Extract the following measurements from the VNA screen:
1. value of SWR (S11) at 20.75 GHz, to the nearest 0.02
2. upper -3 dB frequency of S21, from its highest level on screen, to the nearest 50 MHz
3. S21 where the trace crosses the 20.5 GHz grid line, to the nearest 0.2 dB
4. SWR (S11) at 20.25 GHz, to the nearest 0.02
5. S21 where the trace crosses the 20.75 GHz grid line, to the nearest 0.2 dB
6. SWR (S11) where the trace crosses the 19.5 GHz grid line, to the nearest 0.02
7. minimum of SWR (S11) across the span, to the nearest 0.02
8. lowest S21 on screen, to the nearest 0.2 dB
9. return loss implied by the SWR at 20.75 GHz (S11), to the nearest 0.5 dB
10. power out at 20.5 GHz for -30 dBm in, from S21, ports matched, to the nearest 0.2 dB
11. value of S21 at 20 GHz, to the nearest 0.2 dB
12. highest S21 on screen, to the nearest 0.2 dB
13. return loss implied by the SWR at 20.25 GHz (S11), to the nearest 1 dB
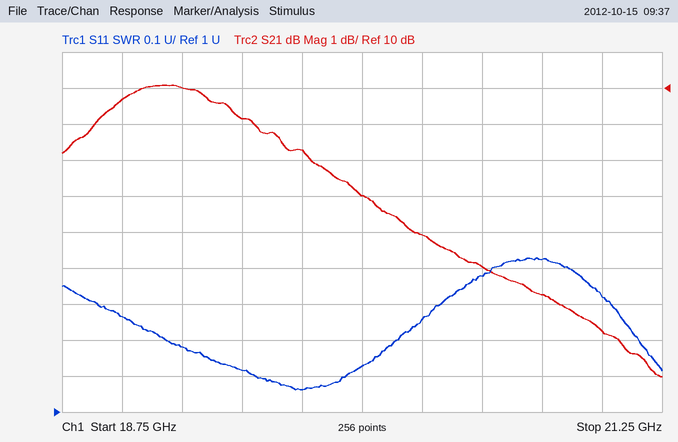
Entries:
1.42
20.00 GHz
5.0 dB
1.26
4.2 dB
1.12
1.06
2.0 dB
15.0 dB
-25.0 dBm
7.0 dB
10.0 dB
19 dB
